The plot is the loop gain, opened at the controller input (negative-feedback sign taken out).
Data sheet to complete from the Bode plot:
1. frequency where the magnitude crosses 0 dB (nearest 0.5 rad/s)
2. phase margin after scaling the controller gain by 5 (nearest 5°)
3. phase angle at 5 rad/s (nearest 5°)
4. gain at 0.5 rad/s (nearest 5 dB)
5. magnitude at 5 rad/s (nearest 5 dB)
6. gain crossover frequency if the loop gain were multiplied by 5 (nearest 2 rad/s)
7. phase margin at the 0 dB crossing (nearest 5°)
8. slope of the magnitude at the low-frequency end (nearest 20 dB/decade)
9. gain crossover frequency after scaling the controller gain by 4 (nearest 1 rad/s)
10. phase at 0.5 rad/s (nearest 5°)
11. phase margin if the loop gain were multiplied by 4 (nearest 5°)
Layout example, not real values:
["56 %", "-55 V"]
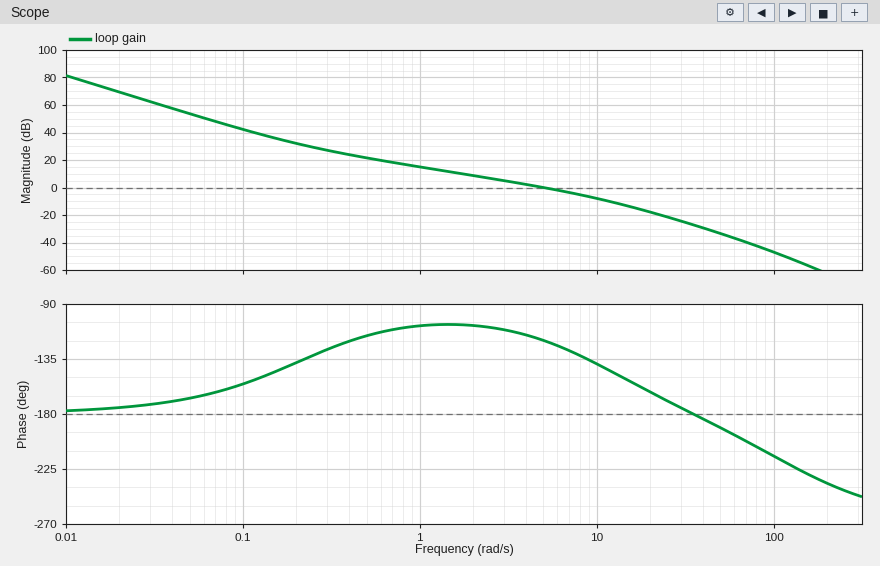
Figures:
["5.0 rad/s", "25°", "-120°", "20 dB", "0 dB", "16 rad/s", "60°", "-40 dB/decade", "14 rad/s", "-115°", "30°"]
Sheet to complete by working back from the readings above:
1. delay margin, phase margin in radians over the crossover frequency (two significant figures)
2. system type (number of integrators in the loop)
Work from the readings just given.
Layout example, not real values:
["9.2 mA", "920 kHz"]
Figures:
["0.21 s", "2"]
